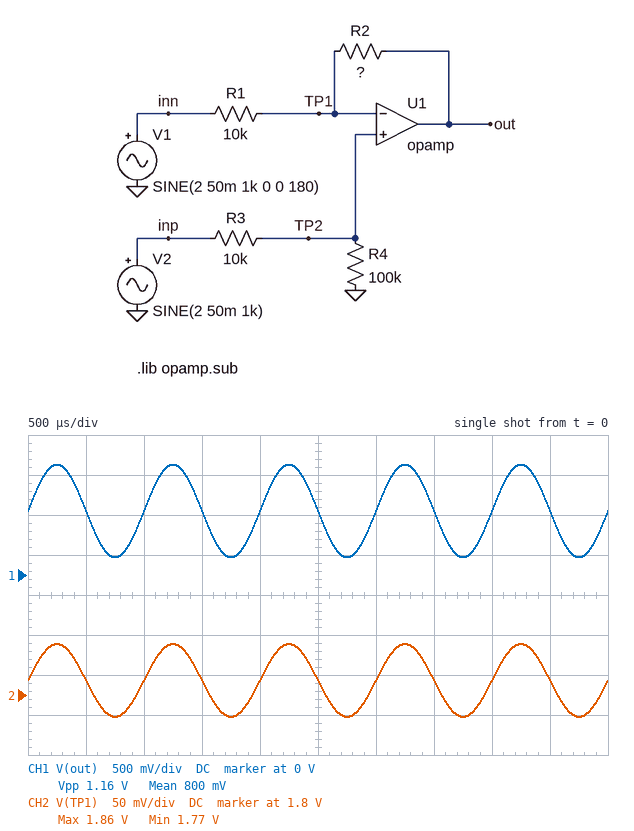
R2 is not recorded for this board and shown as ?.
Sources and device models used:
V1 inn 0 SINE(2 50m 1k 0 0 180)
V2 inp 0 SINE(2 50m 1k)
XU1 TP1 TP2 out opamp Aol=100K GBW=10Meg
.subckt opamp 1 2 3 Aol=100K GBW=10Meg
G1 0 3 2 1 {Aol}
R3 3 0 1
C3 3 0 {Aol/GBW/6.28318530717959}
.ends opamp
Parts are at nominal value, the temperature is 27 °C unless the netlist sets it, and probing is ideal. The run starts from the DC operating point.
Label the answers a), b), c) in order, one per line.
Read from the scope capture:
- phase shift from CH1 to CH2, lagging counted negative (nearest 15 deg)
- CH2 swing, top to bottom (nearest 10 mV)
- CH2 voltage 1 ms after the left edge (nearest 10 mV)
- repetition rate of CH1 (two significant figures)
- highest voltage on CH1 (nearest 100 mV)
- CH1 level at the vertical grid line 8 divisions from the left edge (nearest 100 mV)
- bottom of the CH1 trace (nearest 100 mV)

a) 0 deg
b) 90 mV
c) 1.82 V
d) 1.0 kHz
e) 1.4 V
f) 800 mV
g) 200 mV
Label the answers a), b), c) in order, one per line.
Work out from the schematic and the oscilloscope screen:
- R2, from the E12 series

a) 56 kΩ
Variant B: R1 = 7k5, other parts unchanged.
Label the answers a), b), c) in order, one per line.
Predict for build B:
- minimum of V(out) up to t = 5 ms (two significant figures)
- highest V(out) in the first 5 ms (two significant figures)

a) -300 mV
b) 1.2 V
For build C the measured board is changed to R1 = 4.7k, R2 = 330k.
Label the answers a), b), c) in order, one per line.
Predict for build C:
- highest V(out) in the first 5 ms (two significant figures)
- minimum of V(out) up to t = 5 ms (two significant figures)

a) -4.2 V
b) -18 V
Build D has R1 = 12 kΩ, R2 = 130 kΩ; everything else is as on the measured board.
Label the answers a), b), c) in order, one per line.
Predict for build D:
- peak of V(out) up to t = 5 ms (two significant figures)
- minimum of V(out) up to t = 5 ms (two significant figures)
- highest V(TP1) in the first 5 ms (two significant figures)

a) 930 mV
b) -1.2 V
c) 1.9 V
